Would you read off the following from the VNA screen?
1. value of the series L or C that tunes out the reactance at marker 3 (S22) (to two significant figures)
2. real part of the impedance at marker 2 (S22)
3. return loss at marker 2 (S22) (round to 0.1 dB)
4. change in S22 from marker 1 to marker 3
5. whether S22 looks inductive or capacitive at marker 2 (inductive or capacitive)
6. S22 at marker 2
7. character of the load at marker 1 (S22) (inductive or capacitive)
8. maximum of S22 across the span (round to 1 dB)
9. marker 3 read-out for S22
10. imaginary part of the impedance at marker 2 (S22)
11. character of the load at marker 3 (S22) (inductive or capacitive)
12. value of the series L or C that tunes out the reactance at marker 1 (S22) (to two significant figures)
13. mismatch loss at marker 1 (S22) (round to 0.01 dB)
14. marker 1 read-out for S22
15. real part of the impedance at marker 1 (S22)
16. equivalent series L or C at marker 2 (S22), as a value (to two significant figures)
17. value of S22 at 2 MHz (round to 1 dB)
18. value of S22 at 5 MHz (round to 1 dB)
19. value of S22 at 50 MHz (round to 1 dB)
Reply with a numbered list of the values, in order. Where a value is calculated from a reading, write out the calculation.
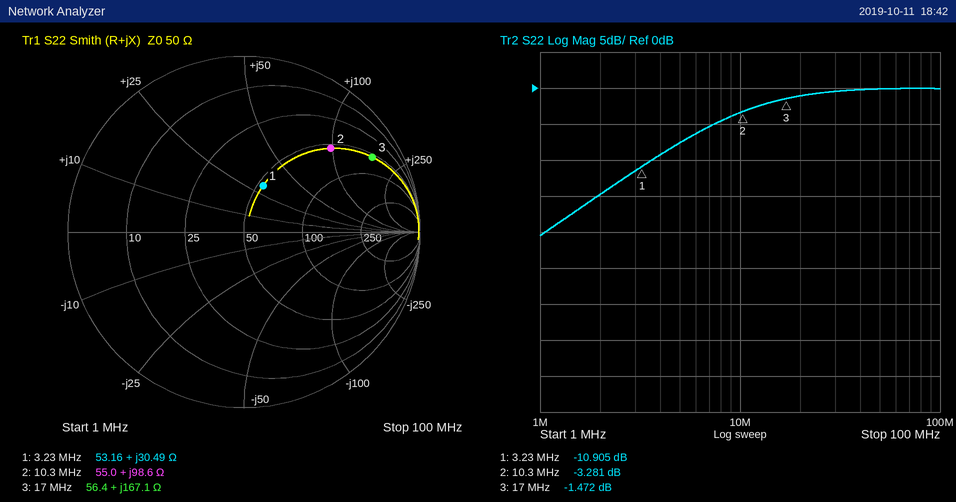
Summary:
1. C = 1/(2π × 17 MHz × 167.1 Ω) ≈ 56 pF
2. 55.0 Ω
3. 3.3 dB
4. -1.472 − (-10.905) = 9.433 dB
5. inductive
6. -3.281 dB
7. inductive
8. 0 dB
9. -1.472 dB
10. +98.6 Ω
11. inductive
12. C = 1/(2π × 3.23 MHz × 30.49 Ω) ≈ 1.6 nF
13. −10 log10(1 − 10^(-10.905/10)) ≈ 0.37 dB
14. -10.905 dB
15. 53.16 Ω
16. L = 98.6 Ω/(2π × 10.3 MHz) ≈ 1.5 µH
17. -15 dB
18. -8 dB
19. 0 dB
